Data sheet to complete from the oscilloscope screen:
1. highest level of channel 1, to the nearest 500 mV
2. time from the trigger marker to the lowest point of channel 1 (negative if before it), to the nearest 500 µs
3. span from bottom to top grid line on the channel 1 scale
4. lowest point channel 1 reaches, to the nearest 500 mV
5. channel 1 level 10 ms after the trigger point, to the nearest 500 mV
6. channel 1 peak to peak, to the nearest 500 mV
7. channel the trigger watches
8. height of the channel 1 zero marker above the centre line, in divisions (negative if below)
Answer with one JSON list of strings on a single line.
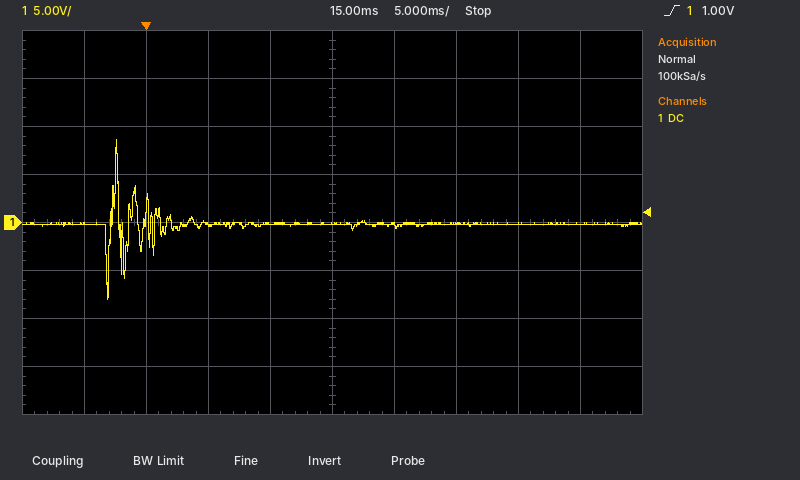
["8.5 V", "-3.0 ms", "40 V", "-8.0 V", "0.0 V", "16.5 V", "channel 1", "0.0 div"]
